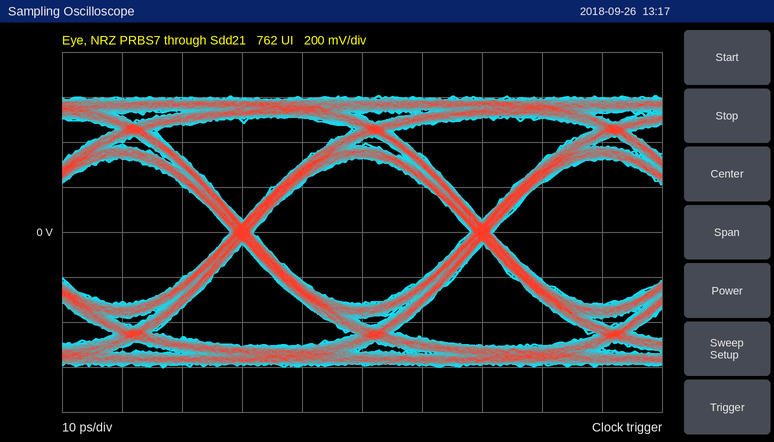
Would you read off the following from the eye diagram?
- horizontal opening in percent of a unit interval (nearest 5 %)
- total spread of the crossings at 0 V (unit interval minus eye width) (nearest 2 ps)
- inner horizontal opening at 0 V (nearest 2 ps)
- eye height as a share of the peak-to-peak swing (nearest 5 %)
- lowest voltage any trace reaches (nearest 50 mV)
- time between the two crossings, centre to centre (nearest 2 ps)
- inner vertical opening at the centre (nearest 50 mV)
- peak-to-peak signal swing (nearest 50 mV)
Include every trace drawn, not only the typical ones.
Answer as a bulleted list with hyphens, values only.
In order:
- 90 %
- 4 ps
- 36 ps
- 55 %
- -600 mV
- 40 ps
- 650 mV
- 1.20 V
